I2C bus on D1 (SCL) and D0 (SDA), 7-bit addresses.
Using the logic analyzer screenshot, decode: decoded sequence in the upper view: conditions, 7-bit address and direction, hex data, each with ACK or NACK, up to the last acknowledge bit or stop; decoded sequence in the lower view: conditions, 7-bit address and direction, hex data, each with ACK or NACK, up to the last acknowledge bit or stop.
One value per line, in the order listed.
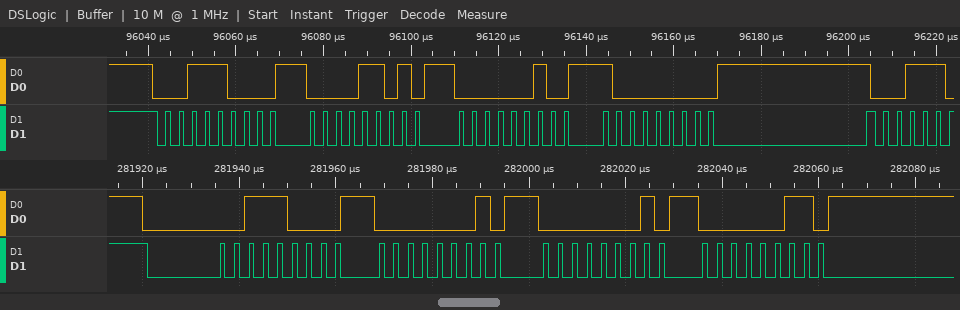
start, address 1C write ACK, 0D ACK, 02 ACK, 80 ACK
start, address 1C write ACK, 01 ACK, 01 ACK, 03 ACK
